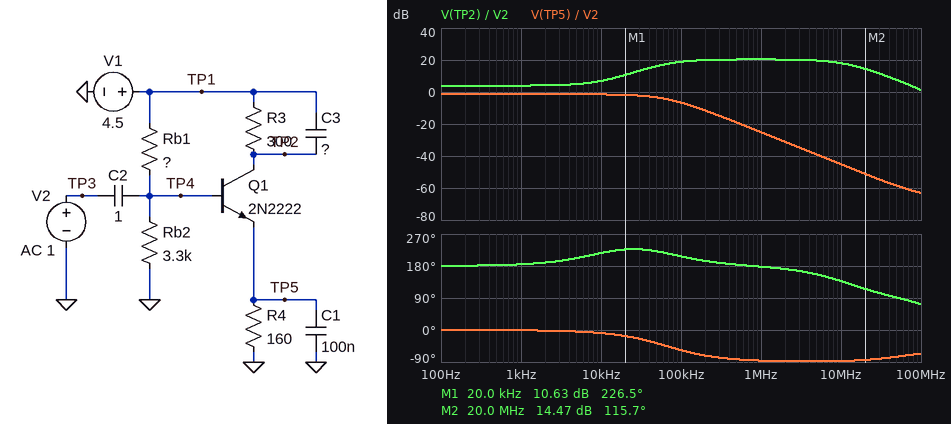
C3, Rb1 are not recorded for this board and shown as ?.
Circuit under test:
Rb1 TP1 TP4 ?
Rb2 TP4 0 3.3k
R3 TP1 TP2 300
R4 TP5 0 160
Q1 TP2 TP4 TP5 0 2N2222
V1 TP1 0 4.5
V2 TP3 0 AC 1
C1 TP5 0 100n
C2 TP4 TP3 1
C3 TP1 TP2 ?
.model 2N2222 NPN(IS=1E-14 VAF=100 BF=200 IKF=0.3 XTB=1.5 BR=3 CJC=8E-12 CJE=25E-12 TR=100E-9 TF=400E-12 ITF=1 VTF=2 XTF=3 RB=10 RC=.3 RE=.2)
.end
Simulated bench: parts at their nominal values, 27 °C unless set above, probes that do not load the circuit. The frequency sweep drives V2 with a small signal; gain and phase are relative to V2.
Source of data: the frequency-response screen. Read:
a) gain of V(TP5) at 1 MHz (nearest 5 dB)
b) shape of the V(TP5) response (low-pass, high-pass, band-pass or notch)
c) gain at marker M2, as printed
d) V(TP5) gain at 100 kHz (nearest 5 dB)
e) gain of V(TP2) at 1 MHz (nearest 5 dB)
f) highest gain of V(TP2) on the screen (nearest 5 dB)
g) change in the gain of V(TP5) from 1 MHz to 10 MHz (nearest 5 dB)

-25 dB
low-pass
14.47 dB
-5 dB
20 dB
20 dB
-20 dB
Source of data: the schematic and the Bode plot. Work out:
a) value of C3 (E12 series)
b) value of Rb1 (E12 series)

39 pF
15 kΩ
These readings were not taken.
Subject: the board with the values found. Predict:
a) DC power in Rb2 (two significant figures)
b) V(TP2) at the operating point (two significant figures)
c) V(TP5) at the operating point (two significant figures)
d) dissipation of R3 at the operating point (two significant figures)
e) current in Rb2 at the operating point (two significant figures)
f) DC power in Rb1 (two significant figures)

190 µW
4.2 V
150 mV
250 µW
240 µA
910 µW
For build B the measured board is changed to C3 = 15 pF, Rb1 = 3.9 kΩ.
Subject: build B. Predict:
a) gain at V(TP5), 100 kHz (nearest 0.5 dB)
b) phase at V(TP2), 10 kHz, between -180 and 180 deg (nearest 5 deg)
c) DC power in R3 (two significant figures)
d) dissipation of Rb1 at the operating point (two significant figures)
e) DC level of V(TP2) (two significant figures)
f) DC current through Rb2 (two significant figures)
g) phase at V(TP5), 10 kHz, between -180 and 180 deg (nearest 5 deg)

-0.5 dB
-135 deg
19 mW
1.6 mW
2.1 V
600 µA
0 deg
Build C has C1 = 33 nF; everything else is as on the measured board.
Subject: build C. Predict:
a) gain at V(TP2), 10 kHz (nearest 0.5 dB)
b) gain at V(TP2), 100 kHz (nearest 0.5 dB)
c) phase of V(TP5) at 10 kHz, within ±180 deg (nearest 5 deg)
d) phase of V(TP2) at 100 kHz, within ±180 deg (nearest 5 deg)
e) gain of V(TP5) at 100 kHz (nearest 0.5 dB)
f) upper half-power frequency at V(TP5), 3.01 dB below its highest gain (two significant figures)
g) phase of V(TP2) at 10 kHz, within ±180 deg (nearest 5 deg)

4.5 dB
14.0 dB
-5 deg
-135 deg
-2.5 dB
200 kHz
-165 deg
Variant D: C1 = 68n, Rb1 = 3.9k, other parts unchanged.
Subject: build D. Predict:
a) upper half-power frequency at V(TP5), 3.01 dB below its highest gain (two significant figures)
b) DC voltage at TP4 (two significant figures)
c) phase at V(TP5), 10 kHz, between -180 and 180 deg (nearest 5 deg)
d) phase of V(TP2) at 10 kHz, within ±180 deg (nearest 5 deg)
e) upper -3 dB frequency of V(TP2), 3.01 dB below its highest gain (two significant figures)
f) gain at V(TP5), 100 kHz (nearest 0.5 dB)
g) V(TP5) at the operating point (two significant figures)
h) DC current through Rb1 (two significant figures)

670 kHz
2.0 V
0 deg
-145 deg
8.8 MHz
-0.5 dB
1.3 V
640 µA
